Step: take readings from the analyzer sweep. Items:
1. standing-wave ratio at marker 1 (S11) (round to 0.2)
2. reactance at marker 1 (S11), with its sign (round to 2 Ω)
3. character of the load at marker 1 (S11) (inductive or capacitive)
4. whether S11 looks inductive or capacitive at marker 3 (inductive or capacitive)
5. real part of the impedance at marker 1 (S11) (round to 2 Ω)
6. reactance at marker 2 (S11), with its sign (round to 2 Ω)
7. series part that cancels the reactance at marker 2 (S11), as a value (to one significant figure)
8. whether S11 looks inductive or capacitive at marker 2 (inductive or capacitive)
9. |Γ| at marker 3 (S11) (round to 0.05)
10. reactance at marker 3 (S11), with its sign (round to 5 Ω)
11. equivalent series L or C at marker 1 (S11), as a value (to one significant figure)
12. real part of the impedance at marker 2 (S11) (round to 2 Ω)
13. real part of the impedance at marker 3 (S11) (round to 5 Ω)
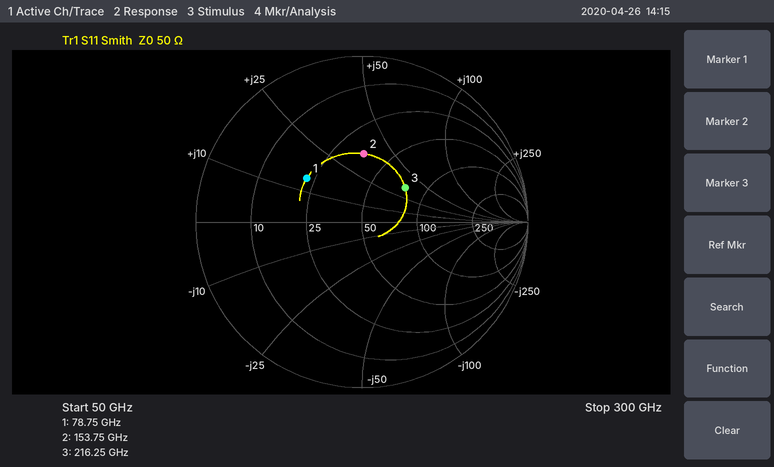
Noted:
2.4
+14 Ω
inductive
inductive
22 Ω
+36 Ω
30 fF
inductive
0.35
+35 Ω
30 pH
36 Ω
75 Ω
